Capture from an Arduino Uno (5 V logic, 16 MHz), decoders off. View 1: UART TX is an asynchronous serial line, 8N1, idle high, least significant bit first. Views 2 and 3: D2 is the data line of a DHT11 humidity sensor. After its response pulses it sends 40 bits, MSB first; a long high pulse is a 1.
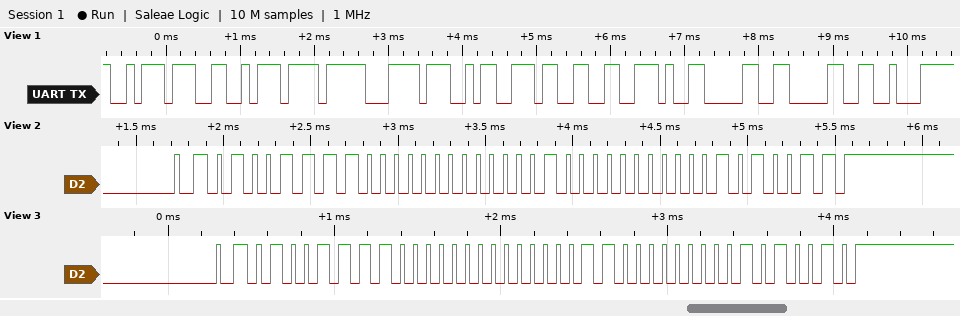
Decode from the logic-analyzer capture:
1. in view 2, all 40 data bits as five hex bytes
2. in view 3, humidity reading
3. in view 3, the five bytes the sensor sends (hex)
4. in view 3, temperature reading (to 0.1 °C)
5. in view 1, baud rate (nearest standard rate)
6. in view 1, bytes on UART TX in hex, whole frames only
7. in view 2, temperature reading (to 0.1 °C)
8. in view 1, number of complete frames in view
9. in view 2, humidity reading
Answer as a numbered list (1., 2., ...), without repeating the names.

1. 4F 00 04 00 53
2. 79 %
3. 4F 00 03 00 52
4. 3.0 °C
5. 9600 baud
6. BA A6 EF BC 9A 33 2E 30 30 E2
7. 4.0 °C
8. 10
9. 79 %
